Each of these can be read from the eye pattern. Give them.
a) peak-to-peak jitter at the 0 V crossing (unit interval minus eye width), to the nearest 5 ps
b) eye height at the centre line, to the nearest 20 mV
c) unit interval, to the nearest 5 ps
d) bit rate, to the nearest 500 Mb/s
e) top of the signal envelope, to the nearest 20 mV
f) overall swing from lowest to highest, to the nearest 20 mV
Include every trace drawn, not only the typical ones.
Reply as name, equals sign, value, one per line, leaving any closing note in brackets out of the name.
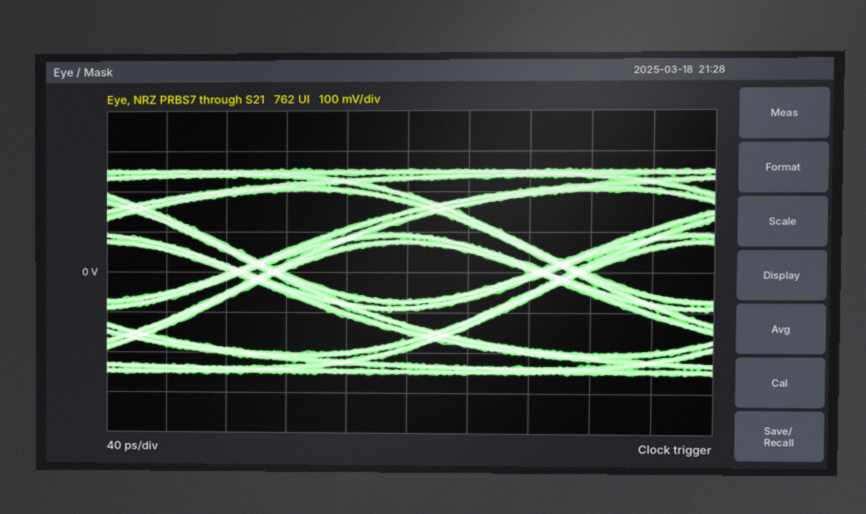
peak-to-peak jitter at the 0 V crossing (unit interval minus eye width), to the nearest 5 ps = 40 ps
eye height at the centre line, to the nearest 20 mV = 140 mV
unit interval, to the nearest 5 ps = 200 ps
bit rate, to the nearest 500 Mb/s = 5.0 Gb/s
top of the signal envelope, to the nearest 20 mV = 260 mV
overall swing from lowest to highest, to the nearest 20 mV = 520 mV
